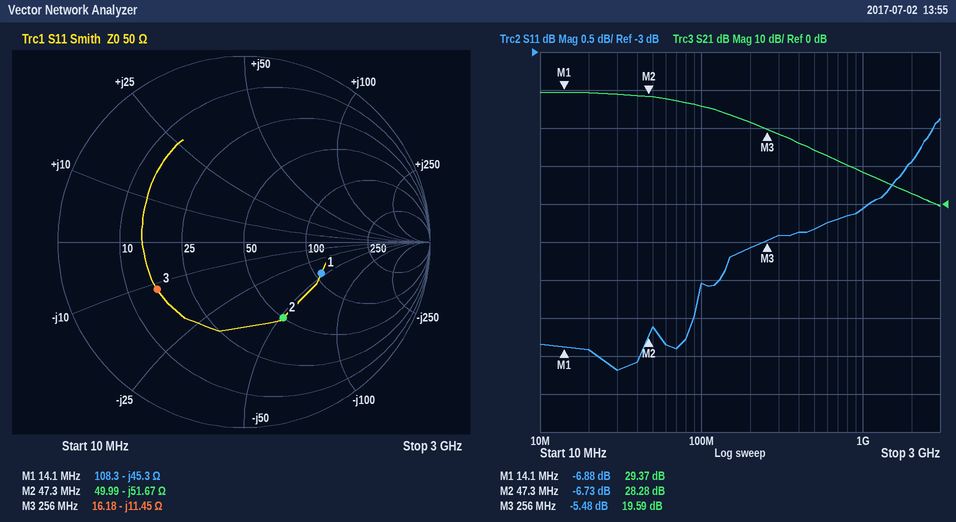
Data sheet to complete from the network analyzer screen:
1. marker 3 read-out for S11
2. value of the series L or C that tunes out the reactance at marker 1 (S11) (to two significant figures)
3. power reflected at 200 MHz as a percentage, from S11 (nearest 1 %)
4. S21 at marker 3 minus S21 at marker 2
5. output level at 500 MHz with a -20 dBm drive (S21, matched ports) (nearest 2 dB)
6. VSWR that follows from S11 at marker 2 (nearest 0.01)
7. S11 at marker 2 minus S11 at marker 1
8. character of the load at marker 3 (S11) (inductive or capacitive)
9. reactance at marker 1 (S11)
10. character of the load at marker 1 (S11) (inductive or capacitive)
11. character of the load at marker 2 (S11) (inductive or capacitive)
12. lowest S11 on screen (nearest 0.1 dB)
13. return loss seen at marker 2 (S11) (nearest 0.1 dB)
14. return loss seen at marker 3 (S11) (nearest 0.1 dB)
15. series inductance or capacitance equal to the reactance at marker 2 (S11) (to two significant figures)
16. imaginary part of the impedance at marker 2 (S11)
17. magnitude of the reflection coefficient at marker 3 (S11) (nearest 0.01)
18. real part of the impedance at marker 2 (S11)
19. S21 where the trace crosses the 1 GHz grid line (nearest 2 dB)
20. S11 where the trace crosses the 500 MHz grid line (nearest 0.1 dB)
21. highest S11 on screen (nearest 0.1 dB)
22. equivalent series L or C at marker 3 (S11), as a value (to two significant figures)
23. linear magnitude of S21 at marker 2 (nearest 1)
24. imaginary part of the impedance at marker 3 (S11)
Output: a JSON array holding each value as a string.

["-5.48 dB", "510 nH", "28 %", "-8.69 dB", "-6 dBm", "2.71", "0.15 dB", "capacitive", "-45.3 Ω", "capacitive", "capacitive", "-7.2 dB", "6.8 dB", "5.5 dB", "65 pF", "-51.67 Ω", "0.53", "49.99 Ω", "8 dB", "-5.3 dB", "-3.9 dB", "54 pF", "26", "-11.45 Ω"]
